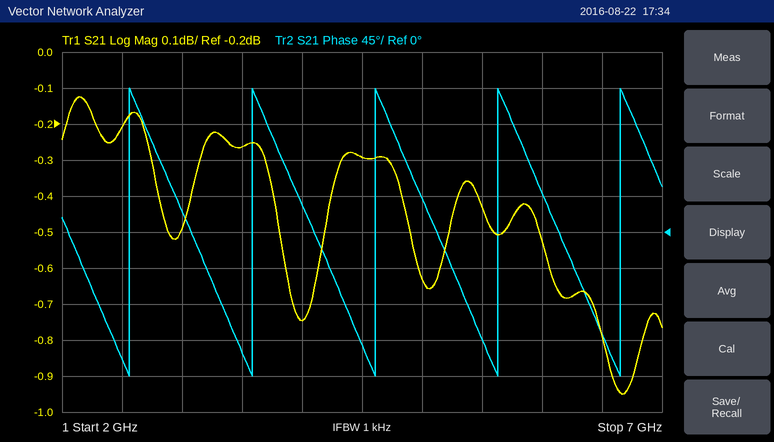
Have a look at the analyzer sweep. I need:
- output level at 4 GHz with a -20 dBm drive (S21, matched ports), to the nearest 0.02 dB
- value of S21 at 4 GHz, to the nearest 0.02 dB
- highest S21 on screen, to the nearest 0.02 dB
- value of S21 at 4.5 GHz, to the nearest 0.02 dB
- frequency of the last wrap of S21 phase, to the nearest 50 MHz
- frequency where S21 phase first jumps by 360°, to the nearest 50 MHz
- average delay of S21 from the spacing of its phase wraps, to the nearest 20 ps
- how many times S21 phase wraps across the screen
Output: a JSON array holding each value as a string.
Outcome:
["-20.74 dBm", "-0.74 dB", "-0.12 dB", "-0.30 dB", "6.65 GHz", "2.55 GHz", "980 ps", "5"]
